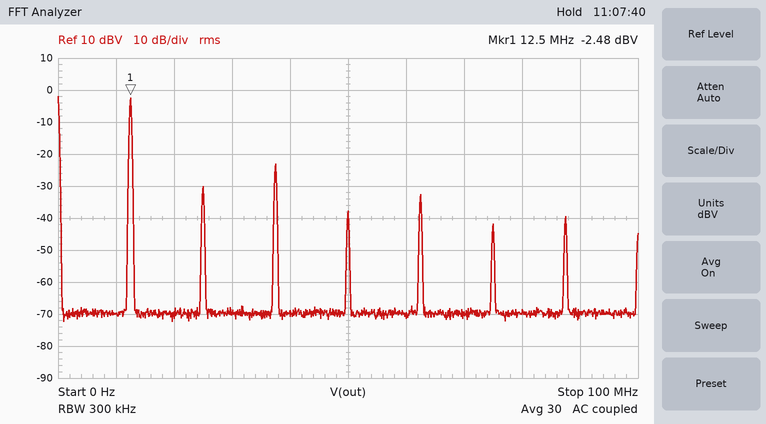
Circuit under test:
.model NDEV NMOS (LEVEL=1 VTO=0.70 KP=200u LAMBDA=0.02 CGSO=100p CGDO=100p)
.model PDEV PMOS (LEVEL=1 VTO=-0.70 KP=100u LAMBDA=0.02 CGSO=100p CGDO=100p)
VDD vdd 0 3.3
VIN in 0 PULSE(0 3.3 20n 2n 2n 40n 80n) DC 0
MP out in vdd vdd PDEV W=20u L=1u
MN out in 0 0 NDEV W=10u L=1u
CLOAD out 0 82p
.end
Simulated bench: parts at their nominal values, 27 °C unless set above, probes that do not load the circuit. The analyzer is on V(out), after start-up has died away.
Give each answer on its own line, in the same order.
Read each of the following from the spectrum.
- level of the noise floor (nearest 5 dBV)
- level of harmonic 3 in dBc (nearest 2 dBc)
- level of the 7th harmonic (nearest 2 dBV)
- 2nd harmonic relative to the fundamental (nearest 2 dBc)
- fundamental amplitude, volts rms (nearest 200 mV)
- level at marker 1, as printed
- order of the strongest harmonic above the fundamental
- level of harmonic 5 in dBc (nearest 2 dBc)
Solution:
-70 dBV
-20 dBc
-40 dBV
-28 dBc
800 mV
-2.48 dBV
3
-30 dBc
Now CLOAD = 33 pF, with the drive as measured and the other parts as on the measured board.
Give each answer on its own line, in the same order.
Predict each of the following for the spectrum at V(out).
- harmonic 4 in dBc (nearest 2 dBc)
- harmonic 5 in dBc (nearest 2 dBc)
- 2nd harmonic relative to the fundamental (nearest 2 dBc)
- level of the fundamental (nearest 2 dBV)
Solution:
-32 dBc
-28 dBc
-26 dBc
2 dBV
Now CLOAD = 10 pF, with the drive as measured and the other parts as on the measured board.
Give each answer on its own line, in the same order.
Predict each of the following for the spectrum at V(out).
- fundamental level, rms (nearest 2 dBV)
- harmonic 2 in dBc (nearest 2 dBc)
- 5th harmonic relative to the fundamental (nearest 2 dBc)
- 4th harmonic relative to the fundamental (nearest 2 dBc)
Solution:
4 dBV
-22 dBc
-18 dBc
-24 dBc
